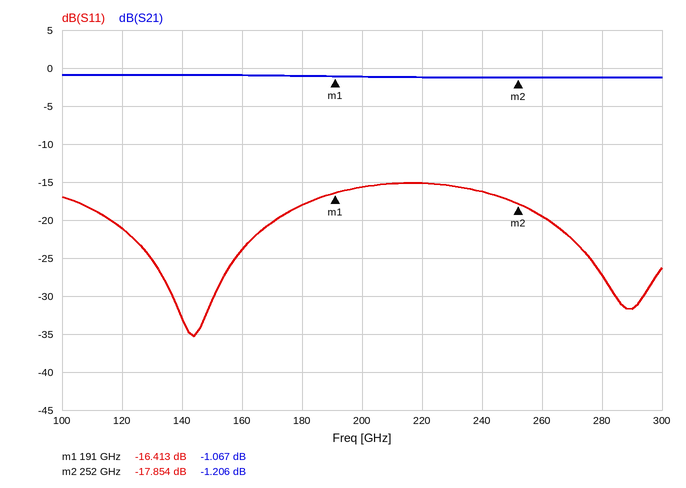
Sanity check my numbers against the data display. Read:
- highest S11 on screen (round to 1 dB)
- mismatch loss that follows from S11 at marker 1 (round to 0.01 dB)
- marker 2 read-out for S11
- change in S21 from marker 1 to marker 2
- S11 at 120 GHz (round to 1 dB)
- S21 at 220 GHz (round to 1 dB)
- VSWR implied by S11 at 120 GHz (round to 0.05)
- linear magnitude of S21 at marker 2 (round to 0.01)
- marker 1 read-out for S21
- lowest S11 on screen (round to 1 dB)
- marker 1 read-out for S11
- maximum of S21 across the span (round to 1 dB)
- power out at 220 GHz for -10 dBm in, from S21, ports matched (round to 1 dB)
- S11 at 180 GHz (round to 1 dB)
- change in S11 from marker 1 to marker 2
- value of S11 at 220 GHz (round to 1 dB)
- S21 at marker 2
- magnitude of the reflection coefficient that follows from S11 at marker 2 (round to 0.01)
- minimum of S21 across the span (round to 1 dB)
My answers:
-15 dB
0.10 dB
-17.854 dB
-0.139 dB
-21 dB
-1 dB
1.20
0.87
-1.067 dB
-35 dB
-16.413 dB
-1 dB
-11 dBm
-18 dB
-1.441 dB
-15 dB
-1.206 dB
0.13
-1 dB
